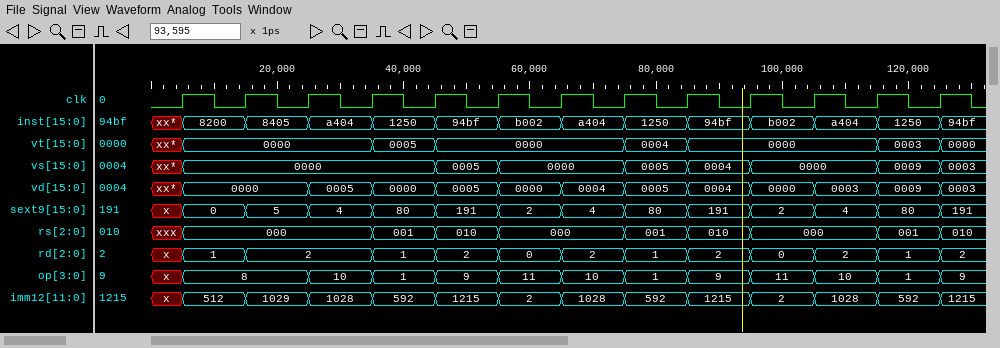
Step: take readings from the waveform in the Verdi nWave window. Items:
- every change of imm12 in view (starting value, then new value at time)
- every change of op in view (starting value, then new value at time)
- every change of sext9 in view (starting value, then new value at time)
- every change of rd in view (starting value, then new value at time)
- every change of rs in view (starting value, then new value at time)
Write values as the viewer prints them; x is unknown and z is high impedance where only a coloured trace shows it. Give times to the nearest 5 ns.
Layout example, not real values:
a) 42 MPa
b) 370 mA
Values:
a) x, 512 at 5 ns, 1029 at 15 ns, 1028 at 25 ns, 592 at 35 ns, 1215 at 45 ns, 2 at 55 ns, 1028 at 65 ns, 592 at 75 ns, 1215 at 85 ns, 2 at 95 ns, 1028 at 105 ns, 592 at 115 ns, 1215 at 125 ns
b) x, 8 at 5 ns, 10 at 25 ns, 1 at 35 ns, 9 at 45 ns, 11 at 55 ns, 10 at 65 ns, 1 at 75 ns, 9 at 85 ns, 11 at 95 ns, 10 at 105 ns, 1 at 115 ns, 9 at 125 ns
c) x, 0 at 5 ns, 5 at 15 ns, 4 at 25 ns, 80 at 35 ns, 191 at 45 ns, 2 at 55 ns, 4 at 65 ns, 80 at 75 ns, 191 at 85 ns, 2 at 95 ns, 4 at 105 ns, 80 at 115 ns, 191 at 125 ns
d) x, 1 at 5 ns, 2 at 15 ns, 1 at 35 ns, 2 at 45 ns, 0 at 55 ns, 2 at 65 ns, 1 at 75 ns, 2 at 85 ns, 0 at 95 ns, 2 at 105 ns, 1 at 115 ns, 2 at 125 ns
e) xxx, 000 at 5 ns, 001 at 35 ns, 010 at 45 ns, 000 at 55 ns, 001 at 75 ns, 010 at 85 ns, 000 at 95 ns, 001 at 115 ns, 010 at 125 ns
